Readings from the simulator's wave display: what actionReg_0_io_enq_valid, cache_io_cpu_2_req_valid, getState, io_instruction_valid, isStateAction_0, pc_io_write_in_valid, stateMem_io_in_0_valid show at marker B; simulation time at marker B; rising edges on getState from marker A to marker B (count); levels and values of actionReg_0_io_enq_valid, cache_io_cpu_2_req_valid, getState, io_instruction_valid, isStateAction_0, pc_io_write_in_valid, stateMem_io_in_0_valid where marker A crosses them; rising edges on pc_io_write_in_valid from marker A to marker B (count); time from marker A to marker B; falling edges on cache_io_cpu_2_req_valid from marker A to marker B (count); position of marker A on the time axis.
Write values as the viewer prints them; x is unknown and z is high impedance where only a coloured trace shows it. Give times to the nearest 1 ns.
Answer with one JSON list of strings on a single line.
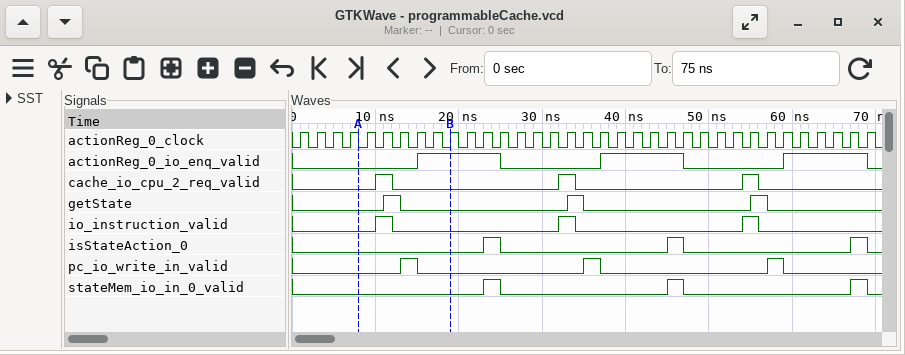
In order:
["actionReg_0_io_enq_valid=1, cache_io_cpu_2_req_valid=0, getState=0, io_instruction_valid=0, isStateAction_0=0, pc_io_write_in_valid=0, stateMem_io_in_0_valid=0", "19 ns", "1", "actionReg_0_io_enq_valid=0, cache_io_cpu_2_req_valid=0, getState=0, io_instruction_valid=0, isStateAction_0=0, pc_io_write_in_valid=0, stateMem_io_in_0_valid=0", "1", "11 ns", "1", "8 ns"]
